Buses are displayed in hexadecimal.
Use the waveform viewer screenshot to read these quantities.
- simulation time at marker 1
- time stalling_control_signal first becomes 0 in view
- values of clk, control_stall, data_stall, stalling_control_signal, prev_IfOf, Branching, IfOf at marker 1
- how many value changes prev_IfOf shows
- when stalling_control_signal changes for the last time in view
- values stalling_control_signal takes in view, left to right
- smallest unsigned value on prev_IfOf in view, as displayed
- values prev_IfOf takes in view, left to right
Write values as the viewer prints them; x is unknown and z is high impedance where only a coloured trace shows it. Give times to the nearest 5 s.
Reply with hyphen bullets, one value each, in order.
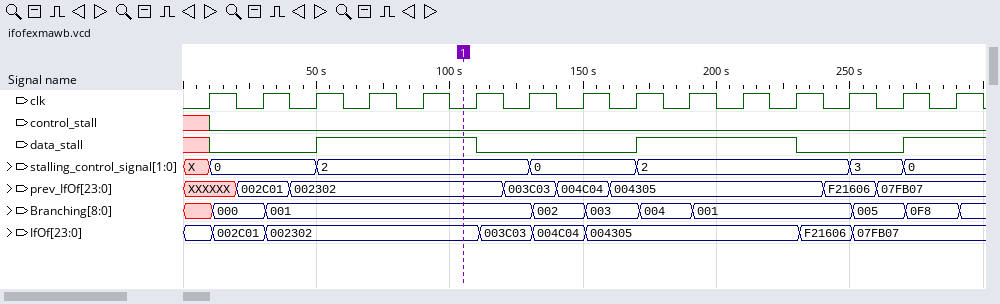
- 105 s
- 10 s
- clk=0, control_stall=0, data_stall=1, stalling_control_signal=2, prev_IfOf=002302, Branching=001, IfOf=002302
- 7
- 270 s
- X, 0, 2, 0, 2, 3, 0
- 002302
- XXXXXX, 002C01, 002302, 003C03, 004C04, 004305, F21606, 07FB07
